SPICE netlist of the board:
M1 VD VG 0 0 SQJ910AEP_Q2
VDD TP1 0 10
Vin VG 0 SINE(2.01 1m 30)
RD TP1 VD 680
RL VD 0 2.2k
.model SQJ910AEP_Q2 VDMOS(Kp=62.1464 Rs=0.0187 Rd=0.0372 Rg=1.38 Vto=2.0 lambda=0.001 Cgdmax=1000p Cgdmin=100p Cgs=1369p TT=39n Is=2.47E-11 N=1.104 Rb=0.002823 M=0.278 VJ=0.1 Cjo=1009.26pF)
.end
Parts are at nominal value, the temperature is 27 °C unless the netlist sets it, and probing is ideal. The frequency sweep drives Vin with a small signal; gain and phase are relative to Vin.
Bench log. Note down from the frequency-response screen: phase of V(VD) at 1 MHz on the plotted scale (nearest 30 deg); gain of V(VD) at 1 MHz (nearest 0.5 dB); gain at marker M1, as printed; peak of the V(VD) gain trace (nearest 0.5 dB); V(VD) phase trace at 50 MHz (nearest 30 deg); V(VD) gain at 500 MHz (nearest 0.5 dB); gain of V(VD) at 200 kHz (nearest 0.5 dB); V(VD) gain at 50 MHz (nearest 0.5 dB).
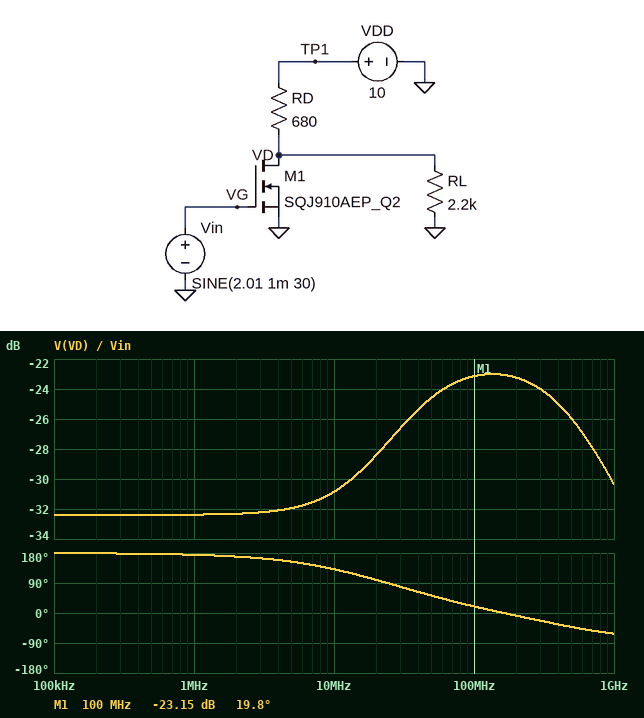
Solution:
180 deg
-32.5 dB
-23.15 dB
-23.0 dB
60 deg
-26.0 dB
-32.5 dB
-24.5 dB
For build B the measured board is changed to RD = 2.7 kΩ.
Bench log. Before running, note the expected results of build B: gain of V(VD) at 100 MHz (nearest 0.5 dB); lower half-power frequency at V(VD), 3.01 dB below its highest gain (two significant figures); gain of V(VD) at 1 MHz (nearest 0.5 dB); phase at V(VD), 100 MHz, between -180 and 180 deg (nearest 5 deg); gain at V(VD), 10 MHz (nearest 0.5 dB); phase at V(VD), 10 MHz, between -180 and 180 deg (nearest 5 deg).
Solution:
-23.5 dB
39 MHz
-44.5 dB
15 deg
-35.5 dB
95 deg
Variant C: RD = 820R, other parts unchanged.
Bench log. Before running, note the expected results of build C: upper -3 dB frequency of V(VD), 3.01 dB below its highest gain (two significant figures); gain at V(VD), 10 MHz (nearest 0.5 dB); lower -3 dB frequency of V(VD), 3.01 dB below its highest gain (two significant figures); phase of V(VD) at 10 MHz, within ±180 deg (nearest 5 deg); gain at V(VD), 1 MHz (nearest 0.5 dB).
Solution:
510 MHz
-32.0 dB
36 MHz
125 deg
-34.0 dB
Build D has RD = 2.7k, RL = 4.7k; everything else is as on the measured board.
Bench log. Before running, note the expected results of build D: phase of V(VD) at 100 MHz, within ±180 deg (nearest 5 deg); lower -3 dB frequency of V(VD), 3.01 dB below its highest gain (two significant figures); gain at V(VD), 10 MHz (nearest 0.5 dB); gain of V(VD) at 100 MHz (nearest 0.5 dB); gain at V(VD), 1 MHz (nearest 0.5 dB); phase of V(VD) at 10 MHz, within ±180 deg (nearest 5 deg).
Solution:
15 deg
39 MHz
-35.5 dB
-23.5 dB
-44.5 dB
95 deg
